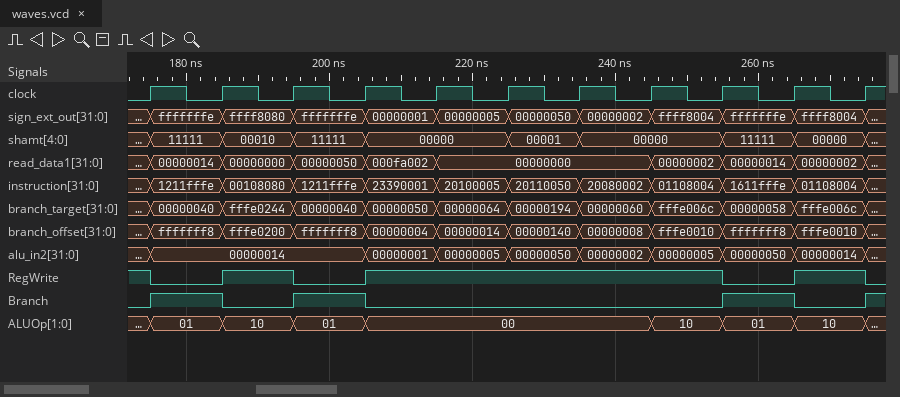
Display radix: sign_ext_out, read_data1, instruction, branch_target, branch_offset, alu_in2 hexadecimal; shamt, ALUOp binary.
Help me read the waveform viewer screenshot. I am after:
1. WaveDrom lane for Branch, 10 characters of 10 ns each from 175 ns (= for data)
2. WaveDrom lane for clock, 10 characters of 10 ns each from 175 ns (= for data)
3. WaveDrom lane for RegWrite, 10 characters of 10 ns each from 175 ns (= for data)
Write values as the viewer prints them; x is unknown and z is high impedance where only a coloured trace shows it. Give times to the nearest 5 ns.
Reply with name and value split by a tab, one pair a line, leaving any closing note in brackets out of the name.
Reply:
WaveDrom lane for Branch, 10 characters of 10 ns each from 175 ns	{name: 'Branch', wave: '1010....10'}
WaveDrom lane for clock, 10 characters of 10 ns each from 175 ns	{name: 'clock', wave: 'p.........'}
WaveDrom lane for RegWrite, 10 characters of 10 ns each from 175 ns	{name: 'RegWrite', wave: '0101....01'}
